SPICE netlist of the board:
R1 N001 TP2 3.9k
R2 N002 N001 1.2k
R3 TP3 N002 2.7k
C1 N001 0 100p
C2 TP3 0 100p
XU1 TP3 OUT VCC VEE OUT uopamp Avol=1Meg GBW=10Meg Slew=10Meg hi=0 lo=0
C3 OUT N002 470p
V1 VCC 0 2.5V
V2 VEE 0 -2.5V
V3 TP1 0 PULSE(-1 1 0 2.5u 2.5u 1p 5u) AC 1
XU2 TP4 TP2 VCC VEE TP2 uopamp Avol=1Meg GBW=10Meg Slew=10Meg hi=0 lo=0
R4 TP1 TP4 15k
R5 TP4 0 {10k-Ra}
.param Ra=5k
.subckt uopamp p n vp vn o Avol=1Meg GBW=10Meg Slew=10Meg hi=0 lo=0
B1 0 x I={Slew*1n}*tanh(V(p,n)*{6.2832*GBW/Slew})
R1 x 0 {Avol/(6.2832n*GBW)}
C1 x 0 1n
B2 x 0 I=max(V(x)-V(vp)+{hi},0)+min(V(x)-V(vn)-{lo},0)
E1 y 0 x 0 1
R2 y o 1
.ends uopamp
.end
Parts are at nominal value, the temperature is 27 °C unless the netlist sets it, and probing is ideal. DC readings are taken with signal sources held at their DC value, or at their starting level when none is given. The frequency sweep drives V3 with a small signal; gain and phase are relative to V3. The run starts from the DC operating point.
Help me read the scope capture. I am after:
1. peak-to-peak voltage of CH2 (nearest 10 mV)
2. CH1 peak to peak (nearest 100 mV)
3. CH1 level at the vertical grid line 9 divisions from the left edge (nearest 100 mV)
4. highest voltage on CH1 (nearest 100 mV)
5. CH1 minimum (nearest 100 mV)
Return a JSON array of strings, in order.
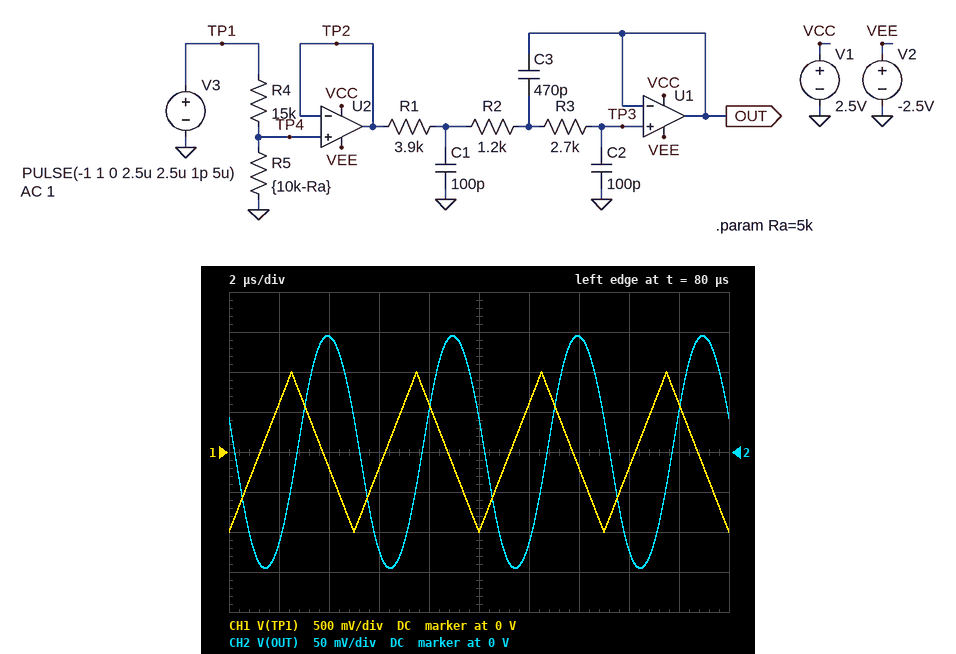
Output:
["290 mV", "2.0 V", "600 mV", "1.0 V", "-1.0 V"]
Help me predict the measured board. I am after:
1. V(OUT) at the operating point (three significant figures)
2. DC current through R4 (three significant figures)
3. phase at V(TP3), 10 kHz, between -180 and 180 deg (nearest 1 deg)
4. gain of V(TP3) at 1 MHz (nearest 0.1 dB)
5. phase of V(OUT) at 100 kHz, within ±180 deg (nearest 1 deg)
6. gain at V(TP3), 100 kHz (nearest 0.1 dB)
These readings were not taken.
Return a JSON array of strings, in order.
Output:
["-250 mV", "50.0 µA", "-4 deg", "-42.5 dB", "-48 deg", "-11.9 dB"]
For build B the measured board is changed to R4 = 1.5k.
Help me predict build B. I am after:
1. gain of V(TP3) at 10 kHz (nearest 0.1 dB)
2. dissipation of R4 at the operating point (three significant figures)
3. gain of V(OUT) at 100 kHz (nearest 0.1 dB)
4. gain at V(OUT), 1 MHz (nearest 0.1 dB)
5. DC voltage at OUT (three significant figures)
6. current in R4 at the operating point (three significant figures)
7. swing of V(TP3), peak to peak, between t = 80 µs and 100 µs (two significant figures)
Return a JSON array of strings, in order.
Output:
["-2.3 dB", "35.5 µW", "-2.1 dB", "-32.8 dB", "-769 mV", "154 µA", "890 mV"]
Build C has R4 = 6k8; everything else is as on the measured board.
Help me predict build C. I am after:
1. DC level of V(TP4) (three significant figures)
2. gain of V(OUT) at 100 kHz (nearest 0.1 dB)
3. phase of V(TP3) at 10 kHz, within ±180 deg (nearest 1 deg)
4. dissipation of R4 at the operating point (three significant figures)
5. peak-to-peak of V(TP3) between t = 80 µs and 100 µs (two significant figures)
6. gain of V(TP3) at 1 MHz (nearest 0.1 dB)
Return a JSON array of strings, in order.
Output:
["-424 mV", "-7.3 dB", "-4 deg", "48.8 µW", "490 mV", "-37.9 dB"]
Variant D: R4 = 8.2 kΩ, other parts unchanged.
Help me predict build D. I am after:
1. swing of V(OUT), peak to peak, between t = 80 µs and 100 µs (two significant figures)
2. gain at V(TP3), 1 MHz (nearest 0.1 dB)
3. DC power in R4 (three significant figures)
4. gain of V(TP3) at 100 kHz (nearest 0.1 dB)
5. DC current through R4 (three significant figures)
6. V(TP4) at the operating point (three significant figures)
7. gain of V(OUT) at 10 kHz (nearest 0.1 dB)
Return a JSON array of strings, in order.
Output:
["440 mV", "-38.9 dB", "47.1 µW", "-8.3 dB", "75.8 µA", "-379 mV", "-8.4 dB"]
